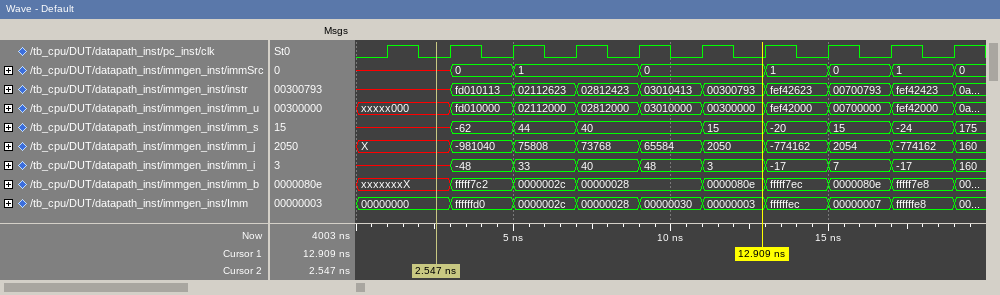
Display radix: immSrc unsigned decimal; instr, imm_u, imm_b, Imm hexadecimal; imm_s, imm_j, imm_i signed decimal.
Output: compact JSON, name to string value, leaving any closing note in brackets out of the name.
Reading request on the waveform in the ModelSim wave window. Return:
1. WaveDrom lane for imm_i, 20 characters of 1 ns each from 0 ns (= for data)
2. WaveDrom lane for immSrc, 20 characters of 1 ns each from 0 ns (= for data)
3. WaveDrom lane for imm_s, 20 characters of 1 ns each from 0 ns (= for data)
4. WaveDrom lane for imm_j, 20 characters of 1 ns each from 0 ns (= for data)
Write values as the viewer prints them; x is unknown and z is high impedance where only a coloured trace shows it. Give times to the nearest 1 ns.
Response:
{"WaveDrom lane for imm_i, 20 characters of 1 ns each from 0 ns": "{name: 'imm_i', wave: 'x..=.=.=.=.=.=.=.=.=', data: '-48 33 40 48 3 -17 7 -17 160'}", "WaveDrom lane for immSrc, 20 characters of 1 ns each from 0 ns": "{name: 'immSrc', wave: 'x..=.=...=...=.=.=.=', data: '0 1 0 1 0 1 0'}", "WaveDrom lane for imm_s, 20 characters of 1 ns each from 0 ns": "{name: 'imm_s', wave: 'x..=.=.=...=.=.=.=.=', data: '-62 44 40 15 -20 15 -24 175'}", "WaveDrom lane for imm_j, 20 characters of 1 ns each from 0 ns": "{name: 'imm_j', wave: '=..=.=.=.=.=.=.=.=.=', data: 'X -981040 75808 73768 65584 2050 -774162 2054 -774162 160'}"}
